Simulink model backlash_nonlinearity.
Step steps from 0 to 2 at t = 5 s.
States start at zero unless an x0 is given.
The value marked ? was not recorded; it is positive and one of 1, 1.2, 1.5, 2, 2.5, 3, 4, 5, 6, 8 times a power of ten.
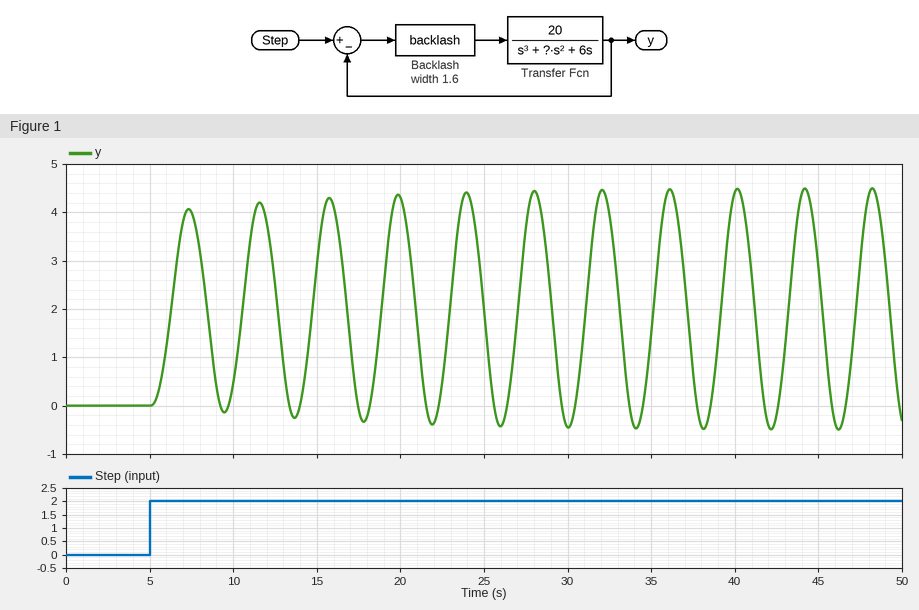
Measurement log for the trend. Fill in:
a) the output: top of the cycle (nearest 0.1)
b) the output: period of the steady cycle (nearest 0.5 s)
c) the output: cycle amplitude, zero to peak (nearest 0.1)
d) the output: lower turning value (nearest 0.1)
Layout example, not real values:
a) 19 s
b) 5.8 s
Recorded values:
a) 4.5
b) 4.0 s
c) 2.5
d) -0.5
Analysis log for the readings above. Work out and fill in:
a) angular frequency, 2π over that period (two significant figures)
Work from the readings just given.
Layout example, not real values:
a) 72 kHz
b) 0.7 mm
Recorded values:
a) 1.6 rad/s
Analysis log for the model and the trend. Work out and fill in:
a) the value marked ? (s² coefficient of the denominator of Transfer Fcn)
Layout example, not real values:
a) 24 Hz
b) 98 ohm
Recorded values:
a) 6
